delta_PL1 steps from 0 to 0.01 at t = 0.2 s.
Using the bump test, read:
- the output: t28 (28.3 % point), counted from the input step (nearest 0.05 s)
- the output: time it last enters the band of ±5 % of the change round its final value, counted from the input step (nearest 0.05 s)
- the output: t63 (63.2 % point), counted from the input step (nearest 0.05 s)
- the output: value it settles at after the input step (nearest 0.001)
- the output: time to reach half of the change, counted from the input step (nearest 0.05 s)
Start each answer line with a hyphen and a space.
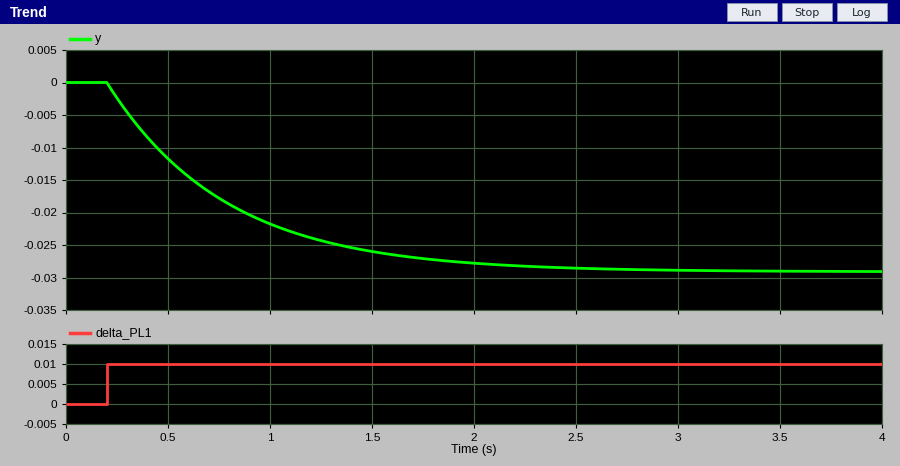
- 0.20 s
- 1.75 s
- 0.60 s
- -0.029
- 0.40 s
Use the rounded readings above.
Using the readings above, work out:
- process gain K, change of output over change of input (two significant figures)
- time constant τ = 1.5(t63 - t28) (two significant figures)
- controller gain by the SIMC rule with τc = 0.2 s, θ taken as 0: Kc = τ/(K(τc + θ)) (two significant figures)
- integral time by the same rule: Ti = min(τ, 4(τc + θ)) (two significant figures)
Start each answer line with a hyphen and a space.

- -2.9
- 0.60 s
- -1.0
- 0.60 s
